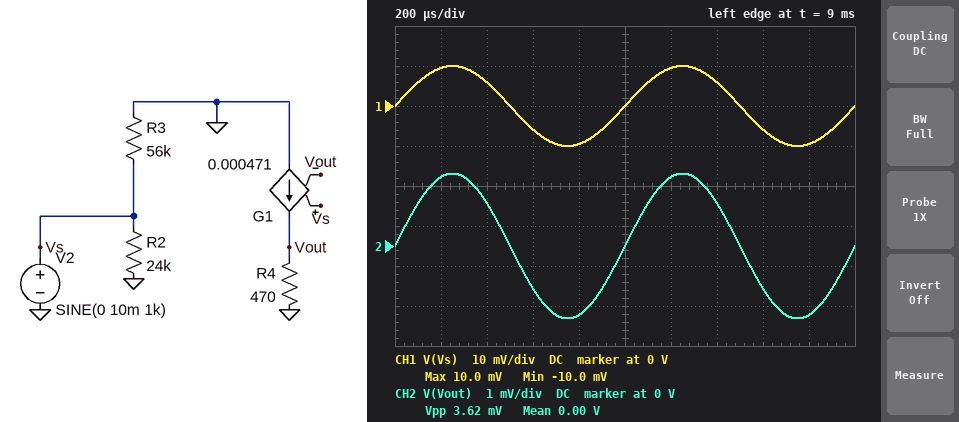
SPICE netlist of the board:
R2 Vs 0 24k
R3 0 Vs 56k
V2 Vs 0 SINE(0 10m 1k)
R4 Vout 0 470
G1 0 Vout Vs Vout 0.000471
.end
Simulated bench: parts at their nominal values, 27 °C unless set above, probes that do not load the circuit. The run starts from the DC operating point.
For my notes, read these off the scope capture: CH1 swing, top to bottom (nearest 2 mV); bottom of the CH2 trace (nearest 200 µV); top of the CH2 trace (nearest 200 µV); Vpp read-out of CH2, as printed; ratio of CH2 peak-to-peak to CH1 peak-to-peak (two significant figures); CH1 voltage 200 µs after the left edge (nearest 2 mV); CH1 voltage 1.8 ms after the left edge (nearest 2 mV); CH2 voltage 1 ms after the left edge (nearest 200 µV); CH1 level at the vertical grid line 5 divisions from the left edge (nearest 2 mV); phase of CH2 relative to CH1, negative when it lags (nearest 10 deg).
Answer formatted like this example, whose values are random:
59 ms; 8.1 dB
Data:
20 mV; -1.8 mV; 1.8 mV; 3.62 mV; 0.18; 10 mV; -10 mV; 0 V; 0 V; 0 deg
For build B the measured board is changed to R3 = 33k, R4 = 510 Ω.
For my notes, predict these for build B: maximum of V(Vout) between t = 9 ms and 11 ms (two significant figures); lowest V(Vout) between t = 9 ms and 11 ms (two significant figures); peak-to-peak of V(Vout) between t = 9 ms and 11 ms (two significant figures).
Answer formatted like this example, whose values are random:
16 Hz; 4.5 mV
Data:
1.9 mV; -1.9 mV; 3.9 mV
